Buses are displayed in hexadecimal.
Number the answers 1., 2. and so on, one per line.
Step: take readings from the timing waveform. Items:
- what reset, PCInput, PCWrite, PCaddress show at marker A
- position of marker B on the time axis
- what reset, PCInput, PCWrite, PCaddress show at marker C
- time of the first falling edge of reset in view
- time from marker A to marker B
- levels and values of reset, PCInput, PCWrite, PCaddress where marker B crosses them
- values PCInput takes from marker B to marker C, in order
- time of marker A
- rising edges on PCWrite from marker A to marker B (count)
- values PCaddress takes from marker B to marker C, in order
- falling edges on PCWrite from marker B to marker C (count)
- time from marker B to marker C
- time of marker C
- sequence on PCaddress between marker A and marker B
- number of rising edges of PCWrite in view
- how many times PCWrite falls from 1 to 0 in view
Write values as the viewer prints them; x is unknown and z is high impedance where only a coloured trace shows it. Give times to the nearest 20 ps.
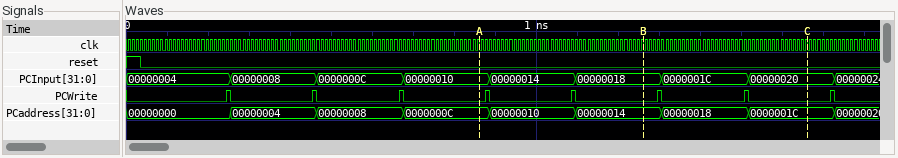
1. reset=0, PCInput=00000010, PCWrite=0, PCaddress=0000000C
2. 1260 ps
3. reset=0, PCInput=00000020, PCWrite=0, PCaddress=0000001C
4. 40 ps
5. 400 ps
6. reset=0, PCInput=00000018, PCWrite=0, PCaddress=00000014
7. 00000018, 0000001C, 00000020
8. 860 ps
9. 2
10. 00000014, 00000018, 0000001C
11. 2
12. 400 ps
13. 1660 ps
14. 0000000C, 00000010, 00000014
15. 8
16. 8
